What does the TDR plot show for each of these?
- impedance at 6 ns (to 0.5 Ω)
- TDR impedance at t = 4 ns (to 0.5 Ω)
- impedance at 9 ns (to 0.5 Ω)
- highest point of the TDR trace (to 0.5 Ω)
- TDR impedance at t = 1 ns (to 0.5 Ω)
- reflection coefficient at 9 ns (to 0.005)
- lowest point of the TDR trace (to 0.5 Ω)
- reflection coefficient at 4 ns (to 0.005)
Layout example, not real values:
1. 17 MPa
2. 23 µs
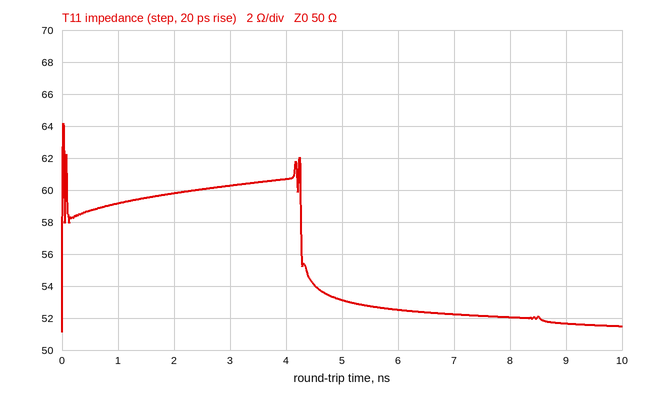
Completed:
1. 52.5 Ω
2. 60.5 Ω
3. 51.5 Ω
4. 64.0 Ω
5. 59.0 Ω
6. +0.015
7. 51.0 Ω
8. +0.095
